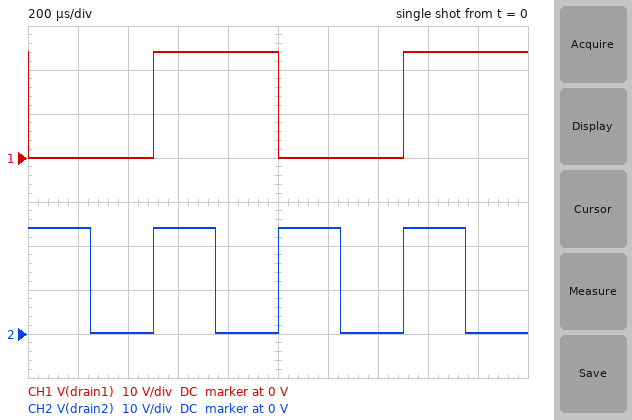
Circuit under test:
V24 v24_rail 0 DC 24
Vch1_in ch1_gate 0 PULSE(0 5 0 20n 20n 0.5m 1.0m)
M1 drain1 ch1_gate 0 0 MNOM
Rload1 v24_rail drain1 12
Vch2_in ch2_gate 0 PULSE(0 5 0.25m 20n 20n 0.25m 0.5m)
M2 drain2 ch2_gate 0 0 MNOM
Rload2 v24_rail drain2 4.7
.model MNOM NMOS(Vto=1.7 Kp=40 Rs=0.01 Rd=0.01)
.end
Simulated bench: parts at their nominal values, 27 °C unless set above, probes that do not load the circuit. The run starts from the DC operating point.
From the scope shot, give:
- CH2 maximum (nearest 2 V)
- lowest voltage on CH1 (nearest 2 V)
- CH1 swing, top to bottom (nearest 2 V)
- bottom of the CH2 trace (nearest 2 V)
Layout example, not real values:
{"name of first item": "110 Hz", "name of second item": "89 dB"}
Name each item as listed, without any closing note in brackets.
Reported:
{"CH2 maximum": "24 V", "lowest voltage on CH1": "0 V", "CH1 swing, top to bottom": "24 V", "bottom of the CH2 trace": "0 V"}
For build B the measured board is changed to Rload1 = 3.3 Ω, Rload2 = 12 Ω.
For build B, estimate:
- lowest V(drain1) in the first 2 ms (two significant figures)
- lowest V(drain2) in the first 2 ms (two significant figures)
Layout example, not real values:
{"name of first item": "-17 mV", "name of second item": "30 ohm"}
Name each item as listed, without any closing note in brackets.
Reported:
{"lowest V(drain1) in the first 2 ms": "200 mV", "lowest V(drain2) in the first 2 ms": "55 mV"}
